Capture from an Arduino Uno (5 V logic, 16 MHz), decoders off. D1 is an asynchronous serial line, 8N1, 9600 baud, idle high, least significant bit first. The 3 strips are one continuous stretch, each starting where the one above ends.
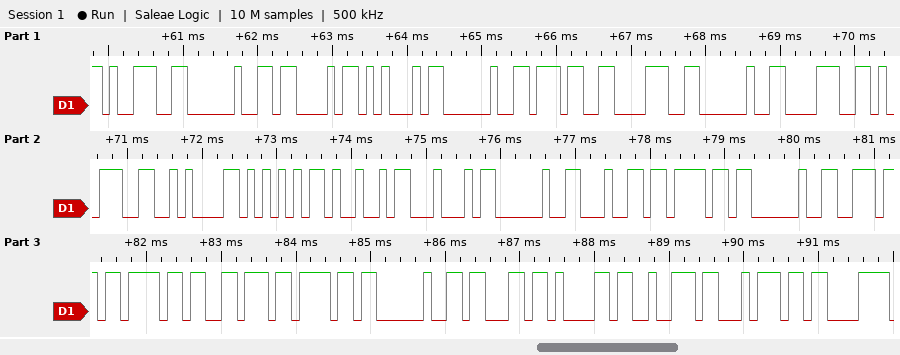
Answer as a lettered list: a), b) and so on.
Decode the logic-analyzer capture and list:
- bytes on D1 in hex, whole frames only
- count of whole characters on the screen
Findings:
a) 39 20 43 45 20 37 38 20 38 39 0A 55 49 44 20 64 6F 20 6E 6F 76 6F 20 63 61 72 74 C3
b) 28
